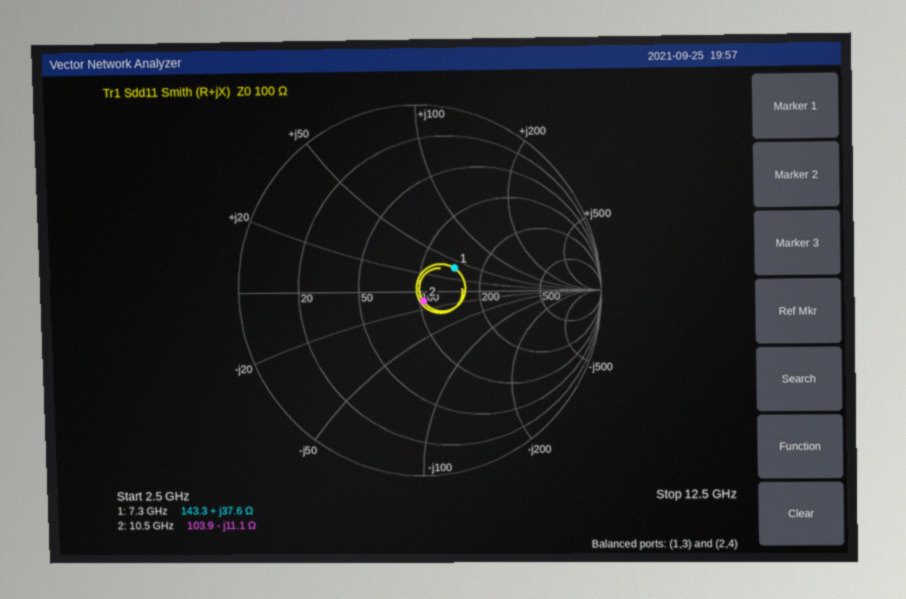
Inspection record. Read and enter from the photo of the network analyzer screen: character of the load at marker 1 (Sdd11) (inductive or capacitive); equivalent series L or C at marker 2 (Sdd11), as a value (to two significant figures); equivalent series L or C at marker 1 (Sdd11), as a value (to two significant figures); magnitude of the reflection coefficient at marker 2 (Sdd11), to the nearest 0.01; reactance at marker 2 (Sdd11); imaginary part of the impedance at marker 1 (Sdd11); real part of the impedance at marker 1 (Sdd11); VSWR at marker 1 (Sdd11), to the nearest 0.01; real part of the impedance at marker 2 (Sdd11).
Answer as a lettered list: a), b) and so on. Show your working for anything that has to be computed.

a) inductive
b) C = 1/(2π × 10.5 GHz × 11.1 Ω) ≈ 1.4 pF
c) L = 37.6 Ω/(2π × 7.3 GHz) ≈ 820 pH
d) 0.06
e) -11.1 Ω
f) +37.6 Ω
g) 143.3 Ω
h) 1.61
i) 103.9 Ω
